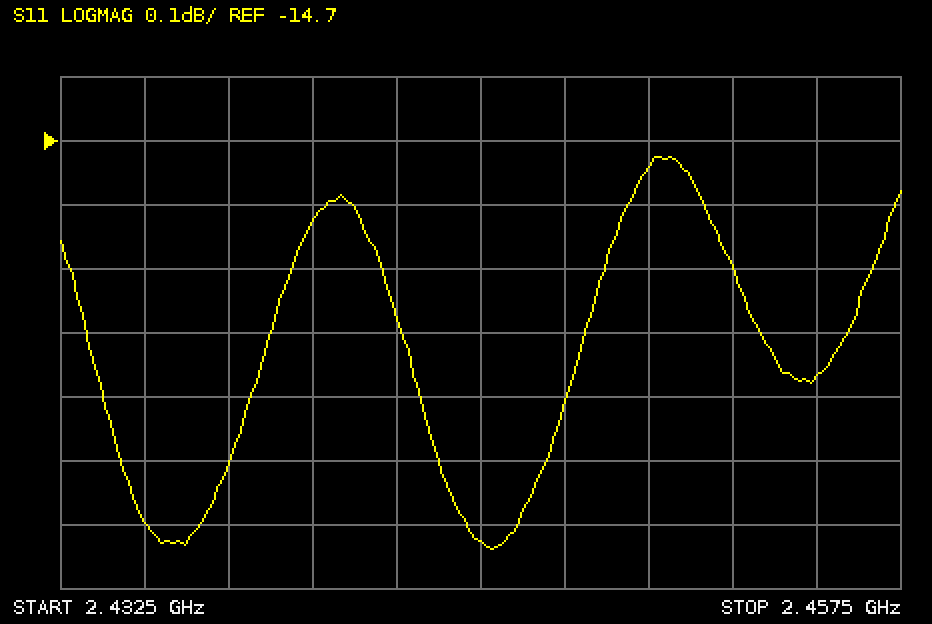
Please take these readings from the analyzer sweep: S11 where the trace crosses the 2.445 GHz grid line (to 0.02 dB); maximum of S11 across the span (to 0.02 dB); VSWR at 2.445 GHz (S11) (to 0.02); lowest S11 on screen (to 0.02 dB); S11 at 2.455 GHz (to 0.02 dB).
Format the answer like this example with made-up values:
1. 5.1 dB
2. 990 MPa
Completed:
1. -15.32 dB
2. -14.72 dB
3. 1.42
4. -15.34 dB
5. -15.06 dB
